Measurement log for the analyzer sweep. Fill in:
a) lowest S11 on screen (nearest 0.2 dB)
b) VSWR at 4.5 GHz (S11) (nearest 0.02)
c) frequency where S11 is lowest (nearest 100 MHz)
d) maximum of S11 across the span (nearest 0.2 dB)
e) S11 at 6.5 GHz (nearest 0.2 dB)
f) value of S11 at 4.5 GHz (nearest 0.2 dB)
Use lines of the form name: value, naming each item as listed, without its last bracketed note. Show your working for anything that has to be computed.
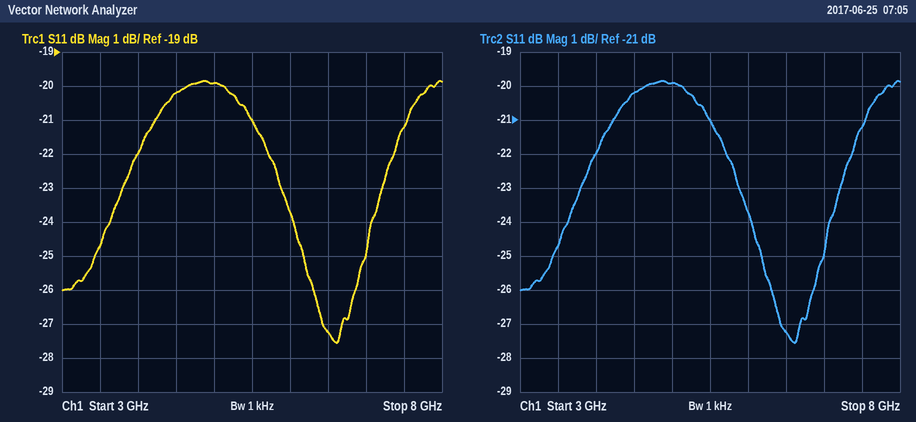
lowest S11 on screen: -27.6 dB
VSWR at 4.5 GHz (S11): |Γ| = 10^(-20.2/20) = 0.0977; VSWR = (1 + 0.0977)/(1 − 0.0977) ≈ 1.22
frequency where S11 is lowest: 6.6 GHz
maximum of S11 across the span: -19.8 dB
S11 at 6.5 GHz: -27.2 dB
value of S11 at 4.5 GHz: -20.2 dB
